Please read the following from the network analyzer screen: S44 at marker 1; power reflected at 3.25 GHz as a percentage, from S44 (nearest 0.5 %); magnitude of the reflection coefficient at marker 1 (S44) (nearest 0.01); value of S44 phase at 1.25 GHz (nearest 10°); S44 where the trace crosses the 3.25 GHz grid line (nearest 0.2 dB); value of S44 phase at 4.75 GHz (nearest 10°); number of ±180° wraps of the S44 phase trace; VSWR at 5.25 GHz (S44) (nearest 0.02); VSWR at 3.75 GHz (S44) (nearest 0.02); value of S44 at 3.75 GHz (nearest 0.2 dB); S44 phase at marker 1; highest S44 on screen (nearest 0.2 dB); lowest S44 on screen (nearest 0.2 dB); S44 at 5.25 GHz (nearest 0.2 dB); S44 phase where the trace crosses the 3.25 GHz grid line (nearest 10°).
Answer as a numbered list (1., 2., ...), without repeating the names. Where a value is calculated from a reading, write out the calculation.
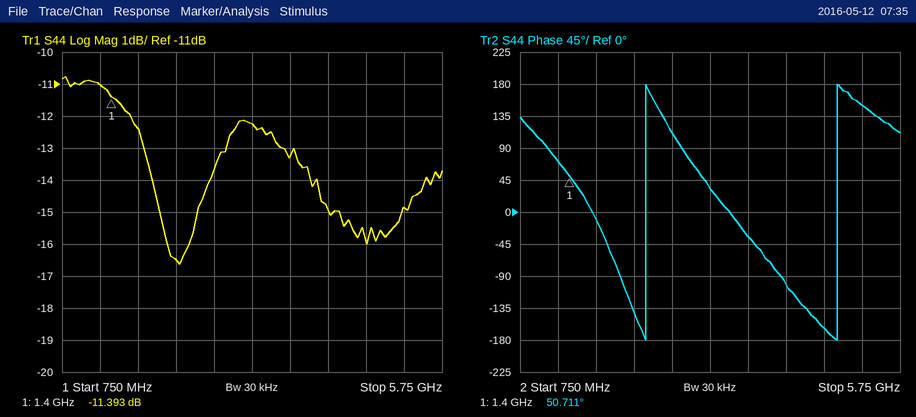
1. -11.393 dB
2. 10^(-12.2/10) ≈ 6.0 %
3. 10^(-11.393/20) ≈ 0.27
4. 70°
5. -12.2 dB
6. -160°
7. 2
8. |Γ| = 10^(-14.8/20) = 0.1820; VSWR = (1 + 0.1820)/(1 − 0.1820) ≈ 1.44
9. |Γ| = 10^(-13.2/20) = 0.2188; VSWR = (1 + 0.2188)/(1 − 0.2188) ≈ 1.56
10. -13.2 dB
11. 50.711°
12. -10.8 dB
13. -16.6 dB
14. -14.8 dB
15. 30°
